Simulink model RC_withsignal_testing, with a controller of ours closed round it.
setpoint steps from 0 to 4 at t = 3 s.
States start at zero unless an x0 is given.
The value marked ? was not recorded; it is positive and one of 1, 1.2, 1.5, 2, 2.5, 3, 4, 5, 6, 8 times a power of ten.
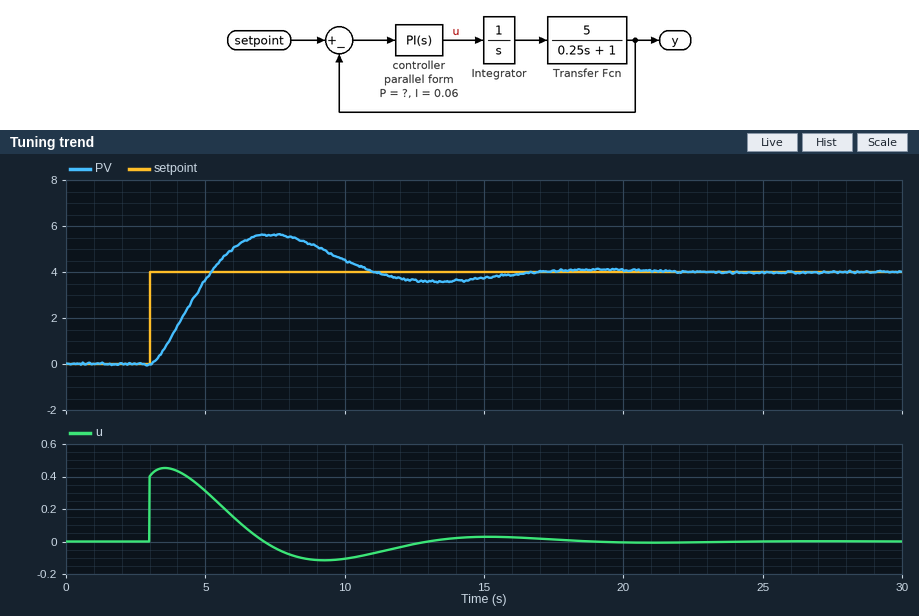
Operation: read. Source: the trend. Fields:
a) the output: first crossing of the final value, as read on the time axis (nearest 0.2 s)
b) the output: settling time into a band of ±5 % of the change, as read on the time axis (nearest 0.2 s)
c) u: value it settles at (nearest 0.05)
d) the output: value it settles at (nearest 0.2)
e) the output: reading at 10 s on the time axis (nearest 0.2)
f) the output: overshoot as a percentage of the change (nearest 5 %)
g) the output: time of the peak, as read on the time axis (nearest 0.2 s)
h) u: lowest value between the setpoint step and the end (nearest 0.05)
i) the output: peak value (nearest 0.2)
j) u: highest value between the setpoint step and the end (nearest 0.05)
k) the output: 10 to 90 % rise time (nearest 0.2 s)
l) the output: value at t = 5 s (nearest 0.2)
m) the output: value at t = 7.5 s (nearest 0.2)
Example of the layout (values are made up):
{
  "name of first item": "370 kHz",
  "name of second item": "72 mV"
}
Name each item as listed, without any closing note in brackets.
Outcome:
{
  "the output: first crossing of the final value, as read on the time axis": "5.2 s",
  "the output: settling time into a band of ±5 % of the change, as read on the time axis": "15.4 s",
  "u: value it settles at": "0.00",
  "the output: value it settles at": "4.0",
  "the output: reading at 10 s on the time axis": "4.6",
  "the output: overshoot as a percentage of the change": "40 %",
  "the output: time of the peak, as read on the time axis": "7.4 s",
  "u: lowest value between the setpoint step and the end": "-0.10",
  "the output: peak value": "5.6",
  "u: highest value between the setpoint step and the end": "0.45",
  "the output: 10 to 90 % rise time": "1.6 s",
  "the output: value at t = 5 s": "3.6",
  "the output: value at t = 7.5 s": "5.6"
}
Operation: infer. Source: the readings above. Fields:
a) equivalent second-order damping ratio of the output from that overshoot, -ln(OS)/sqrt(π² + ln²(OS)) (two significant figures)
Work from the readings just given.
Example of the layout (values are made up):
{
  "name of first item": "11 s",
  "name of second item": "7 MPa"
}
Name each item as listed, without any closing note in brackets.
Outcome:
{
  "equivalent second-order damping ratio of the output from that overshoot, -ln(OS)/sqrt(π² + ln²(OS))": "0.28"
}
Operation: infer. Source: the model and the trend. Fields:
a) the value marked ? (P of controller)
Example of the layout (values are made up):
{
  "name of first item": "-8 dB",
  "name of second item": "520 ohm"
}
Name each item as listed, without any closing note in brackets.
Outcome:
{
  "the value marked ?": "0.1"
}
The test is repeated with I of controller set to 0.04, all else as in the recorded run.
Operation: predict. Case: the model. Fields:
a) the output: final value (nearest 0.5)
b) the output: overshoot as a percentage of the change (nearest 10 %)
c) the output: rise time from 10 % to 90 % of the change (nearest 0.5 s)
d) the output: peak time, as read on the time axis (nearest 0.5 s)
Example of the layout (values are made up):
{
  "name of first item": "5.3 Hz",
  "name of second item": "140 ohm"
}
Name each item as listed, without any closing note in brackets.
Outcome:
{
  "the output: final value": "4.0",
  "the output: overshoot as a percentage of the change": "30 %",
  "the output: rise time from 10 % to 90 % of the change": "2.0 s",
  "the output: peak time, as read on the time axis": "8.0 s"
}
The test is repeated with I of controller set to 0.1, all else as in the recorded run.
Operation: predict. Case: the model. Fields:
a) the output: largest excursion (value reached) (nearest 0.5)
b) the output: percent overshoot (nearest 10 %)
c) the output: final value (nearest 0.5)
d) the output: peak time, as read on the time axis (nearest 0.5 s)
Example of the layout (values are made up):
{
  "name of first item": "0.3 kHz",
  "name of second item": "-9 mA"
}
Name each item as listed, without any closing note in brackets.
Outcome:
{
  "the output: largest excursion (value reached)": "6.0",
  "the output: percent overshoot": "50 %",
  "the output: final value": "4.0",
  "the output: peak time, as read on the time axis": "6.5 s"
}
